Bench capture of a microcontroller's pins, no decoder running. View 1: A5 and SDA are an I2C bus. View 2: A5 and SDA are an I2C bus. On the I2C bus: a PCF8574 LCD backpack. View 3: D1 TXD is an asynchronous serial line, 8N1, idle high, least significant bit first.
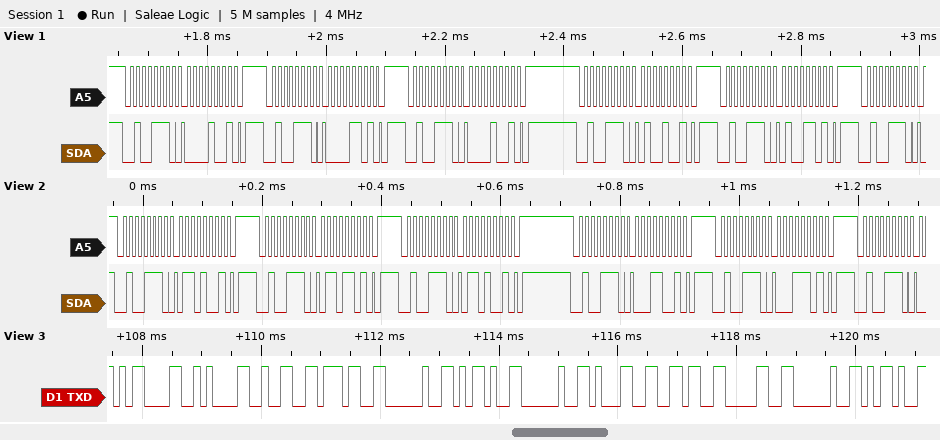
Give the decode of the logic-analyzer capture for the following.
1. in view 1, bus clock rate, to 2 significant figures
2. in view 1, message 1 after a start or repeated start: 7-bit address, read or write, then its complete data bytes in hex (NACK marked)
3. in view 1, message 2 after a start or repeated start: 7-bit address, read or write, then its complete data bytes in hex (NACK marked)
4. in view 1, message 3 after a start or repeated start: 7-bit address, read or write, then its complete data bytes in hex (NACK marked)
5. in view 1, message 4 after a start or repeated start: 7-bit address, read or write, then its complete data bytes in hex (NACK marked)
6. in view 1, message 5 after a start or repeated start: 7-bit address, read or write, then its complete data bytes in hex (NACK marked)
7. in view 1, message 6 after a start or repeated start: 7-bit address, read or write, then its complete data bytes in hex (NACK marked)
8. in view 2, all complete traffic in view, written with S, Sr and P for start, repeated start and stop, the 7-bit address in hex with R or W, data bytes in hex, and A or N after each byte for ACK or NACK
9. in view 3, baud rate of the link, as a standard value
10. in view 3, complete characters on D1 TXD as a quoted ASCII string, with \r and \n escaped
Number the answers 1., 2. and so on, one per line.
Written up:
1. 100 kHz
2. 0x27 write: 09
3. 0x27 write: 0D
4. 0x27 write: 09
5. 0x27 write: 49
6. 0x27 write: 4D
7. 0x27 write
8. S 27W A 69 A P S 27W A 6D A P S 27W A 69 A P S 27W A 19 A P S 27W A 1D A P S 27W A
9. 9600 baud
10. "\r\n27 - 160 -"
